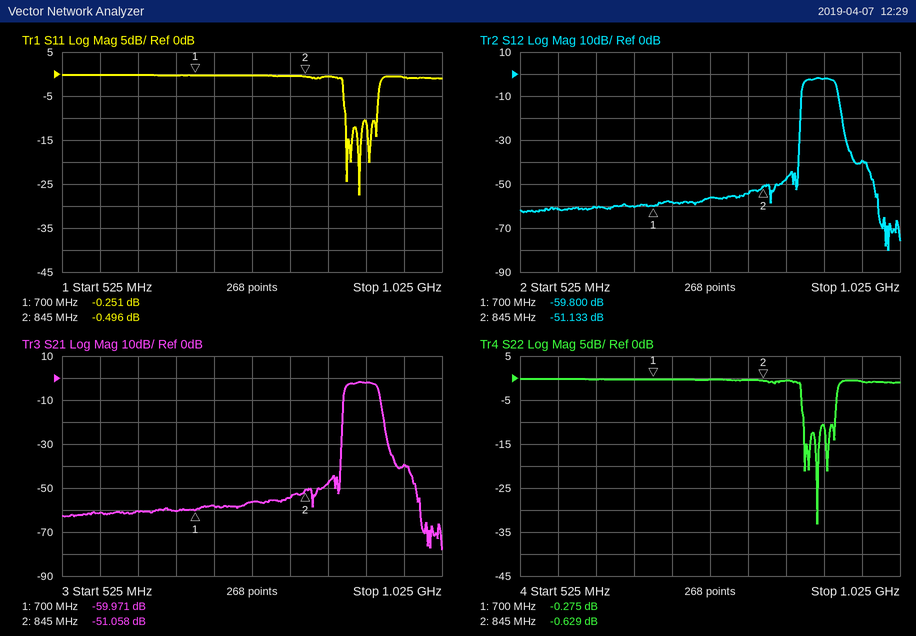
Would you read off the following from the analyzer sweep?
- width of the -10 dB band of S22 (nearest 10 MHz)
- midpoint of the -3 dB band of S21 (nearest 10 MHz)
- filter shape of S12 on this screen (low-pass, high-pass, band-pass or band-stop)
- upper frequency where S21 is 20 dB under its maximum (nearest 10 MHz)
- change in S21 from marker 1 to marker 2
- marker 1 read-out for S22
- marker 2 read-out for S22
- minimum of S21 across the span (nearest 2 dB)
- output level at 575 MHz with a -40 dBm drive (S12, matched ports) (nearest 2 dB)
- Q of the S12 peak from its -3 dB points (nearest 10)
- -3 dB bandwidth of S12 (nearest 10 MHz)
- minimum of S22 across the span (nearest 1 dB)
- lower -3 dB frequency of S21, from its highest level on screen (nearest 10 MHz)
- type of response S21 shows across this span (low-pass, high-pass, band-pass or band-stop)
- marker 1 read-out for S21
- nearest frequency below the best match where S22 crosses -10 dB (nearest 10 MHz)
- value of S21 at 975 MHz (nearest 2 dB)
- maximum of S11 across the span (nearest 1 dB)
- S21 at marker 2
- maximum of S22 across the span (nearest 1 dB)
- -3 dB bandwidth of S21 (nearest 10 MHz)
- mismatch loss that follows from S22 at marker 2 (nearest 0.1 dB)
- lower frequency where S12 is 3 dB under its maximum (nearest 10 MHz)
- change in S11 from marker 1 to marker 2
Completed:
40 MHz
920 MHz
band-pass
950 MHz
8.913 dB
-0.275 dB
-0.629 dB
-78 dB
-102 dBm
20
40 MHz
-33 dB
900 MHz
band-pass
-59.971 dB
900 MHz
-40 dB
0 dB
-51.058 dB
0 dB
40 MHz
8.7 dB
900 MHz
-0.245 dB
